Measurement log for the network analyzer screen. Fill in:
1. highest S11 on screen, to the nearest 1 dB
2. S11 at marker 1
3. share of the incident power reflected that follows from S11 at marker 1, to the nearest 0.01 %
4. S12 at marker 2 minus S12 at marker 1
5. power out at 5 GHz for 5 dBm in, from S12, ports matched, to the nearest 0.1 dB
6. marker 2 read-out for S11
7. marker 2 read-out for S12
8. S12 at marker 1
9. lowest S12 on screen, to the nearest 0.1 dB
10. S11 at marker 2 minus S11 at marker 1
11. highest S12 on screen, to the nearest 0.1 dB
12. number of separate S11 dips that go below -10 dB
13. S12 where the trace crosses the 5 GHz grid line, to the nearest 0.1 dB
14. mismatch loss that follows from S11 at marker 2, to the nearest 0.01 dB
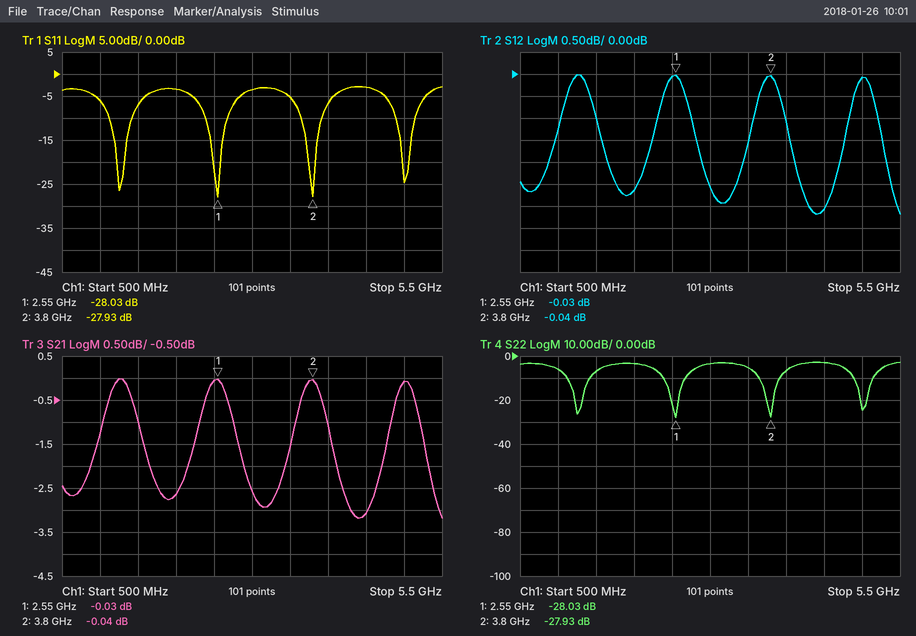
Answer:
-3 dB
-28.03 dB
0.16 %
-0.01 dB
4.9 dBm
-27.93 dB
-0.04 dB
-0.03 dB
-3.2 dB
0.10 dB
0.0 dB
4
-0.1 dB
0.01 dB
